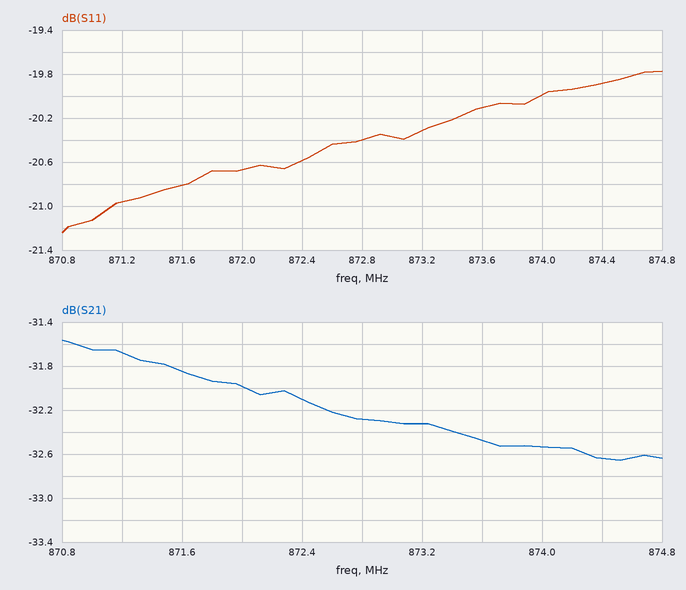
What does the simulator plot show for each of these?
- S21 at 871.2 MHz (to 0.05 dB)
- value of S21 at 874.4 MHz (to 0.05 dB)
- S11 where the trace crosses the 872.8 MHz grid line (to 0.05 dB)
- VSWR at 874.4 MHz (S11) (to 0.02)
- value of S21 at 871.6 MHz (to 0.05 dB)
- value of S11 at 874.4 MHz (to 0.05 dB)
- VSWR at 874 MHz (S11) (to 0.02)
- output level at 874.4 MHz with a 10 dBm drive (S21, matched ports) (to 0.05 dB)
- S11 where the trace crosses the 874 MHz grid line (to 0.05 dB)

-31.70 dB
-32.65 dB
-20.40 dB
1.22
-31.85 dB
-19.90 dB
1.22
-22.65 dBm
-20.00 dB
